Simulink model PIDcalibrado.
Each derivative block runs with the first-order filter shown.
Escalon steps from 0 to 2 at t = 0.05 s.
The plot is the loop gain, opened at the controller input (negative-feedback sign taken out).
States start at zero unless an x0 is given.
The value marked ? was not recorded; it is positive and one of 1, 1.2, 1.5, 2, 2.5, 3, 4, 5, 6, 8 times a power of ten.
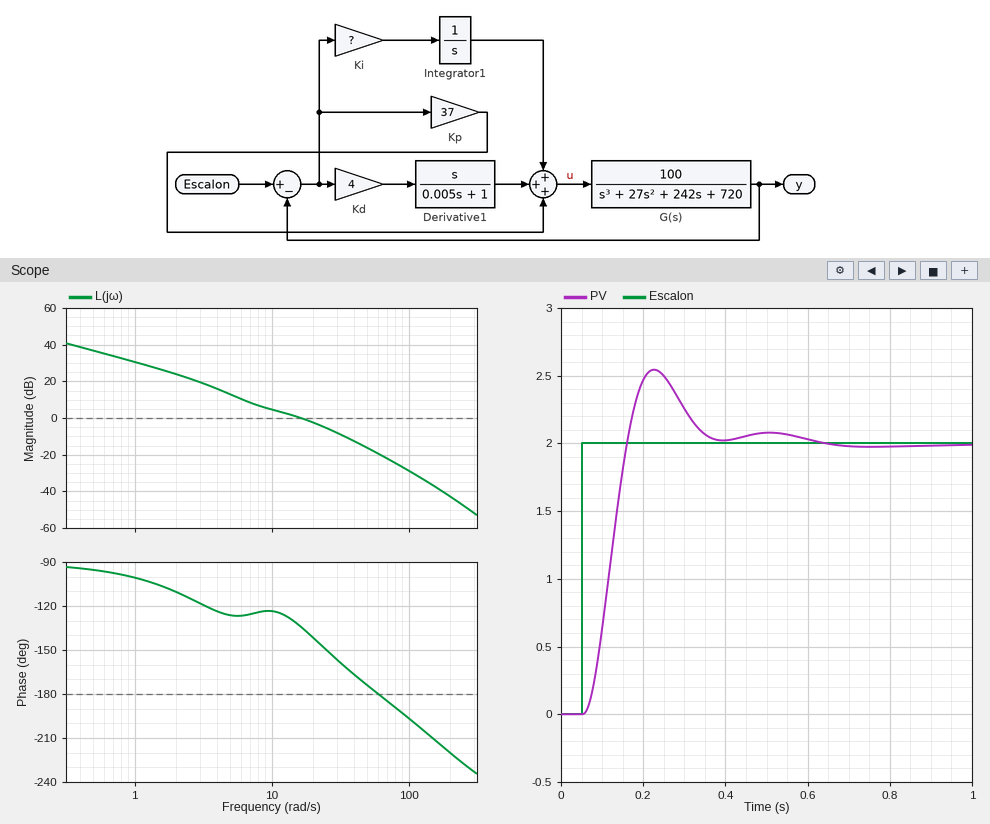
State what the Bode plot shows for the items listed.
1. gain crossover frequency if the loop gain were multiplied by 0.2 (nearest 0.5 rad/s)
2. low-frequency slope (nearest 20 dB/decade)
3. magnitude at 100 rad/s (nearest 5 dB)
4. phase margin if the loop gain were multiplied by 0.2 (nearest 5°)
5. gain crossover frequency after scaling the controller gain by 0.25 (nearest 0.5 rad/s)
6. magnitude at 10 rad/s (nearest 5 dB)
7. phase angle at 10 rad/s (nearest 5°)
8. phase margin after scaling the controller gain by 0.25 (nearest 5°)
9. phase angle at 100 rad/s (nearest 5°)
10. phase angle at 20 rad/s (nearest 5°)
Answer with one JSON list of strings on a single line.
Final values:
["4.5 rad/s", "-20 dB/decade", "-30 dB", "55°", "5.5 rad/s", "5 dB", "-125°", "55°", "-195°", "-140°"]
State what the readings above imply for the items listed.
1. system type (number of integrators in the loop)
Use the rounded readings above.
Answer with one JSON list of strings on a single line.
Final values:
["1"]
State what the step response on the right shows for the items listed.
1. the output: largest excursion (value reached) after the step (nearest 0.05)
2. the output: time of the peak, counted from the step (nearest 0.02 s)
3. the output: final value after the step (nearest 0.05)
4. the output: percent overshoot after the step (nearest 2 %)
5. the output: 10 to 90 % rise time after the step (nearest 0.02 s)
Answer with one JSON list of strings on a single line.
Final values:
["2.55", "0.18 s", "2.00", "28 %", "0.08 s"]
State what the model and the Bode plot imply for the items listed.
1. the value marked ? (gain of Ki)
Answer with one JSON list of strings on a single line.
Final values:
["250"]
